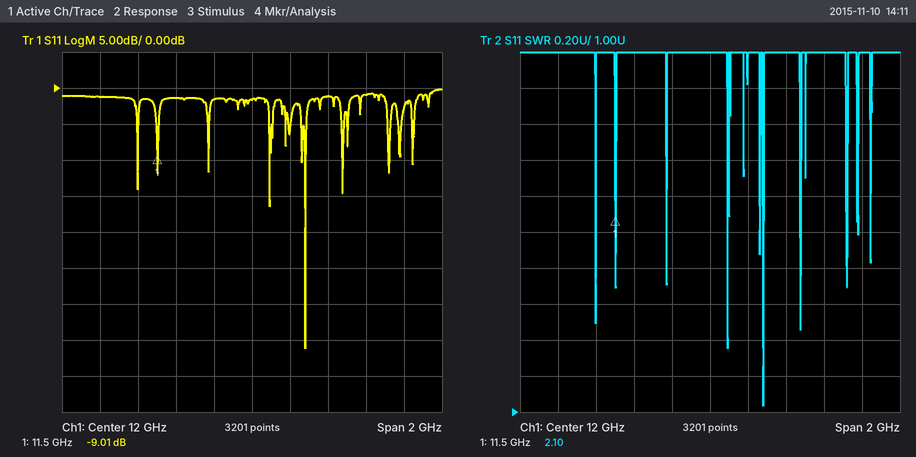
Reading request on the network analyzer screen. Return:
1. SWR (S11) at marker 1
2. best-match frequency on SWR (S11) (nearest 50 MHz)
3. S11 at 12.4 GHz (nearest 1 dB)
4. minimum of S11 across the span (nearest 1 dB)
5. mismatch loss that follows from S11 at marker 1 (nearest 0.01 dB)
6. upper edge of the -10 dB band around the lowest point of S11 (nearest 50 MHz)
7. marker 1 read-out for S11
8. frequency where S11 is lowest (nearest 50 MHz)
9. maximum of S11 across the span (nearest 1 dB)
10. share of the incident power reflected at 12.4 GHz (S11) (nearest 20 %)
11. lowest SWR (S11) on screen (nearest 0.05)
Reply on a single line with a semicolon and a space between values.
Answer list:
2.10; 12.30 GHz; -1 dB; -36 dB; 0.58 dB; 12.30 GHz; -9.01 dB; 12.30 GHz; 0 dB; 80 %; 1.05
